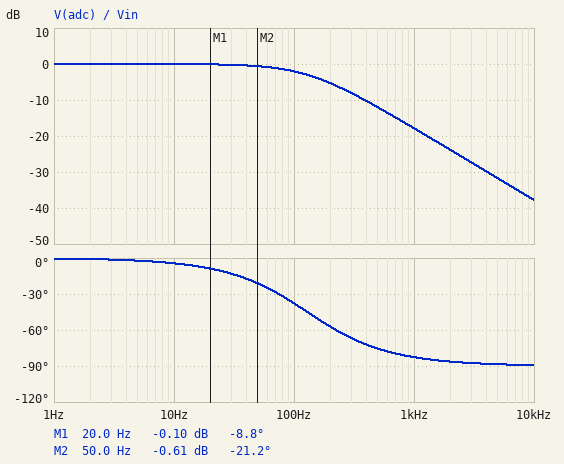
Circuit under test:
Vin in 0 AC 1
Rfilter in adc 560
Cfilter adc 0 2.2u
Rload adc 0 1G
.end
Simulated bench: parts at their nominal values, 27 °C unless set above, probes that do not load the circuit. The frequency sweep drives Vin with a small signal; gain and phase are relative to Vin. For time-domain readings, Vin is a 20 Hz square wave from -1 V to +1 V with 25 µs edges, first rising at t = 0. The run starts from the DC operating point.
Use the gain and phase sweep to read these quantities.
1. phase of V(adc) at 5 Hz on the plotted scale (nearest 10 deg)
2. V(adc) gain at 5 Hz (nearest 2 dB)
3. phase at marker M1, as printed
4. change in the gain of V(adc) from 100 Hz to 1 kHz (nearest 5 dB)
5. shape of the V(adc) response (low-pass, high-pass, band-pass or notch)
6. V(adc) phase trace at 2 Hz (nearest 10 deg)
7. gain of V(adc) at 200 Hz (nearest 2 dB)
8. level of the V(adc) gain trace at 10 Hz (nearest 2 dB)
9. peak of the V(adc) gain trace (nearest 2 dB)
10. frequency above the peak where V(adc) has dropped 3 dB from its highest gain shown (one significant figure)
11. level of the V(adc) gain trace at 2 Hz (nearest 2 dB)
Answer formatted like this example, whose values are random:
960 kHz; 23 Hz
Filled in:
0 deg; 0 dB; -8.8 deg; -15 dB; low-pass; 0 deg; -6 dB; 0 dB; 0 dB; 100 Hz; 0 dB
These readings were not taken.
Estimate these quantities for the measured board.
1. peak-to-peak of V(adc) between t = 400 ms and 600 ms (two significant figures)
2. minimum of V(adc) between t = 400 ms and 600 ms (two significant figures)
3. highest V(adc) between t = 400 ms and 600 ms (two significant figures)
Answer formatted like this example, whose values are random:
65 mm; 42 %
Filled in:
2.0 V; -1.0 V; 1.0 V
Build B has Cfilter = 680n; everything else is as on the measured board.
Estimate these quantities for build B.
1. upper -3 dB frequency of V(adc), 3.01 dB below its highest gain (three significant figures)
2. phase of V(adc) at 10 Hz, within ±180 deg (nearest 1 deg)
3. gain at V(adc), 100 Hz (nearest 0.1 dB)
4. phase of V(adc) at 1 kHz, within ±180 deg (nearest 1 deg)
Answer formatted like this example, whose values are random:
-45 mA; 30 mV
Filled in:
418 Hz; -1 deg; -0.2 dB; -67 deg
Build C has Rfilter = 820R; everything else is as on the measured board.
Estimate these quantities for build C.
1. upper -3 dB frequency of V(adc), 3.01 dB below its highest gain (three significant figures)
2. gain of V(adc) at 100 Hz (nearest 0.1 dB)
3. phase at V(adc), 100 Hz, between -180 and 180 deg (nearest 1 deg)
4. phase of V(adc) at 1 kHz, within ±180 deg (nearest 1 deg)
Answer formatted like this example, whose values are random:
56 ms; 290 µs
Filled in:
88.2 Hz; -3.6 dB; -49 deg; -85 deg
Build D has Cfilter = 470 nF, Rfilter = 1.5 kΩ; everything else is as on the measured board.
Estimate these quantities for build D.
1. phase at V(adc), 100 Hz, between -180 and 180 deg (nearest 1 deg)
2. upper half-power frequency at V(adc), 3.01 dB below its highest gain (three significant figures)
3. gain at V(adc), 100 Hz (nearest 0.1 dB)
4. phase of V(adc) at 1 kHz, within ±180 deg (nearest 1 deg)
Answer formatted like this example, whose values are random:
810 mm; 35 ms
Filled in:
-24 deg; 226 Hz; -0.8 dB; -77 deg
